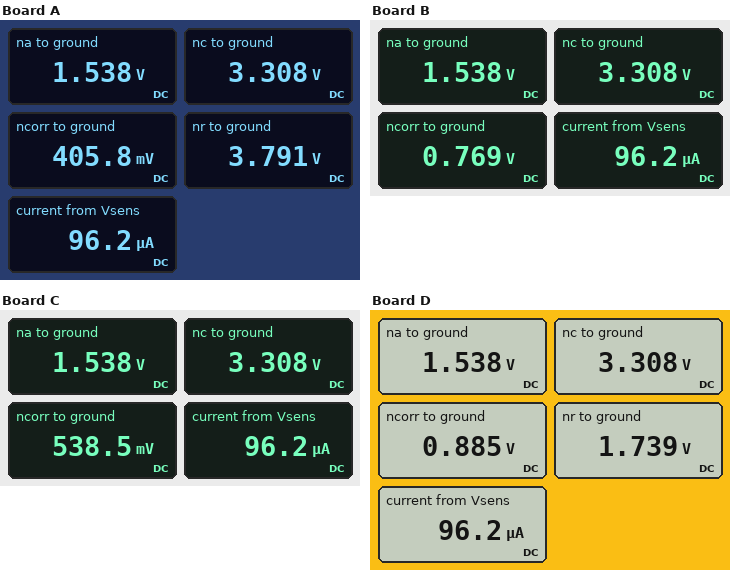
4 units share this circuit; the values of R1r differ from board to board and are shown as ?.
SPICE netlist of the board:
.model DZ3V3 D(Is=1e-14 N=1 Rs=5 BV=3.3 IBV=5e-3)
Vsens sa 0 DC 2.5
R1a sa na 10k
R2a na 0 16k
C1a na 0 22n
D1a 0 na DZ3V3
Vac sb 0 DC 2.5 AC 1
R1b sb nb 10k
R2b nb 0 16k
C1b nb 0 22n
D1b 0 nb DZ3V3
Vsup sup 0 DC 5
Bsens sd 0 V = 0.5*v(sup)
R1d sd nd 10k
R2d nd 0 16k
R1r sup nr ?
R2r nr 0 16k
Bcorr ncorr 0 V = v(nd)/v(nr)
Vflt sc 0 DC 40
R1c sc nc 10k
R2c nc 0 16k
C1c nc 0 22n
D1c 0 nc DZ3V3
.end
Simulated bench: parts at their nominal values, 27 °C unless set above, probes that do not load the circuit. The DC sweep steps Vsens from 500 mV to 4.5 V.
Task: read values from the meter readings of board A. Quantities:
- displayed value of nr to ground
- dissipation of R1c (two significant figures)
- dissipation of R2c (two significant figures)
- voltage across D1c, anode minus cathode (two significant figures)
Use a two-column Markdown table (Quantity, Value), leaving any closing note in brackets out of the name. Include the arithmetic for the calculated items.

| Quantity | Value |
|---|---|
| displayed value of nr to ground | 3.791 V |
| dissipation of R1c | (40 V - 3.308 V)^2 / 10 kΩ = 130 mW |
| dissipation of R2c | (3.308 V)^2 / 16 kΩ = 680 µW |
| voltage across D1c, anode minus cathode | 0 V - 3.308 V = -3.3 V |
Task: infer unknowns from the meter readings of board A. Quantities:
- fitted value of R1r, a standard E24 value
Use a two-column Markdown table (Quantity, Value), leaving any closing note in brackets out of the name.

| Quantity | Value |
|---|---|
| fitted value of R1r, a standard E24 value | 5.1 kΩ |
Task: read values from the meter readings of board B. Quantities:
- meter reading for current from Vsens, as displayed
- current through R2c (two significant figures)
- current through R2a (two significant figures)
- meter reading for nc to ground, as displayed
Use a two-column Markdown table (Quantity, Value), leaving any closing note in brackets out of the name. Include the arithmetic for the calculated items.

| Quantity | Value |
|---|---|
| meter reading for current from Vsens, as displayed | 96.2 µA |
| current through R2c | (3.308 V) / 16 kΩ = 210 µA |
| current through R2a | (1.538 V) / 16 kΩ = 96 µA |
| meter reading for nc to ground, as displayed | 3.308 V |
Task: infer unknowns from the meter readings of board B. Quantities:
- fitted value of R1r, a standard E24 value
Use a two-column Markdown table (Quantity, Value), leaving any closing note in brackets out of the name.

| Quantity | Value |
|---|---|
| fitted value of R1r, a standard E24 value | 24 kΩ |
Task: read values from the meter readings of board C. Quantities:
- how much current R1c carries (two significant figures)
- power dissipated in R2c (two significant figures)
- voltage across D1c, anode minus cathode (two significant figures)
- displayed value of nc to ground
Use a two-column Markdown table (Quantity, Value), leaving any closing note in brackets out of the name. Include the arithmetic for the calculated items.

| Quantity | Value |
|---|---|
| how much current R1c carries | (40 V - 3.308 V) / 10 kΩ = 3.7 mA |
| power dissipated in R2c | (3.308 V)^2 / 16 kΩ = 680 µW |
| voltage across D1c, anode minus cathode | 0 V - 3.308 V = -3.3 V |
| displayed value of nc to ground | 3.308 V |
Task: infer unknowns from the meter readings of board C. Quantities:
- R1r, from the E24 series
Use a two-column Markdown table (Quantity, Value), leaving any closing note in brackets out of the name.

| Quantity | Value |
|---|---|
| R1r, from the E24 series | 12 kΩ |
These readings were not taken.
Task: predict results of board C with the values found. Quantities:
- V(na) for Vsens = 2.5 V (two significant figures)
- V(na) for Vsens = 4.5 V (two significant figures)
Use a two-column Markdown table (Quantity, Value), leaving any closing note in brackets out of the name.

| Quantity | Value |
|---|---|
| V(na) for Vsens = 2.5 V | 1.5 V |
| V(na) for Vsens = 4.5 V | 2.8 V |
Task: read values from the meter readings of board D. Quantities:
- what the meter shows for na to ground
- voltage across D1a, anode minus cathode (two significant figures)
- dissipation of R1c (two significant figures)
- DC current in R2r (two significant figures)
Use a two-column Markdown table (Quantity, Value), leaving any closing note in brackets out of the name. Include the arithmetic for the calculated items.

| Quantity | Value |
|---|---|
| what the meter shows for na to ground | 1.538 V |
| voltage across D1a, anode minus cathode | 0 V - 1.538 V = -1.5 V |
| dissipation of R1c | (40 V - 3.308 V)^2 / 10 kΩ = 130 mW |
| DC current in R2r | (1.739 V) / 16 kΩ = 110 µA |
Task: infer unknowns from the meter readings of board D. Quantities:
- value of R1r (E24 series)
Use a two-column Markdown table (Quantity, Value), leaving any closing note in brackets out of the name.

| Quantity | Value |
|---|---|
| value of R1r | 30 kΩ |
